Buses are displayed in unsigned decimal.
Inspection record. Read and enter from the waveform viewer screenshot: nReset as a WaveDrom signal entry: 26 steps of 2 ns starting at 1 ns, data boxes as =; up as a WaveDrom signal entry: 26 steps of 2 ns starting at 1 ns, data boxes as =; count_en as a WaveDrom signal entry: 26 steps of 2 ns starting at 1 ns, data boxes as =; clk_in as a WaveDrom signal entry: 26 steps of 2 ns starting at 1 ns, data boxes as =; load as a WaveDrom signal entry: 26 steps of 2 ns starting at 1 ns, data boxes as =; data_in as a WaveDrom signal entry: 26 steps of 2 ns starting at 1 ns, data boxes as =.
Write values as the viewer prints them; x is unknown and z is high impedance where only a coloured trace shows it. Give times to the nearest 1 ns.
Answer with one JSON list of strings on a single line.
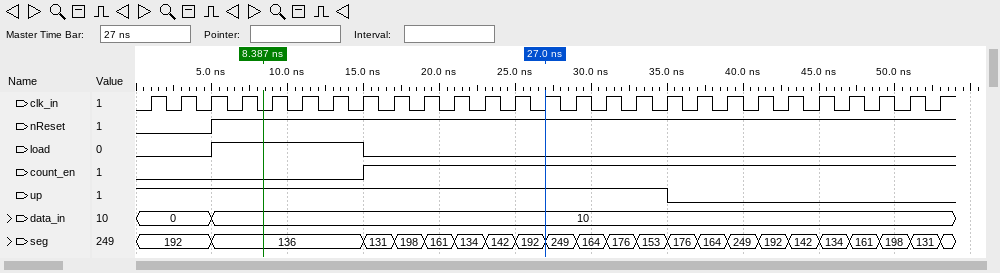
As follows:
["{name: 'nReset', wave: '0.1.......................'}", "{name: 'up', wave: '1................0........'}", "{name: 'count_en', wave: '0......1..................'}", "{name: 'clk_in', wave: 'p.........................'}", "{name: 'load', wave: '0.1....0..................'}", "{name: 'data_in', wave: '=.=.......................', data: '0 10'}"]
